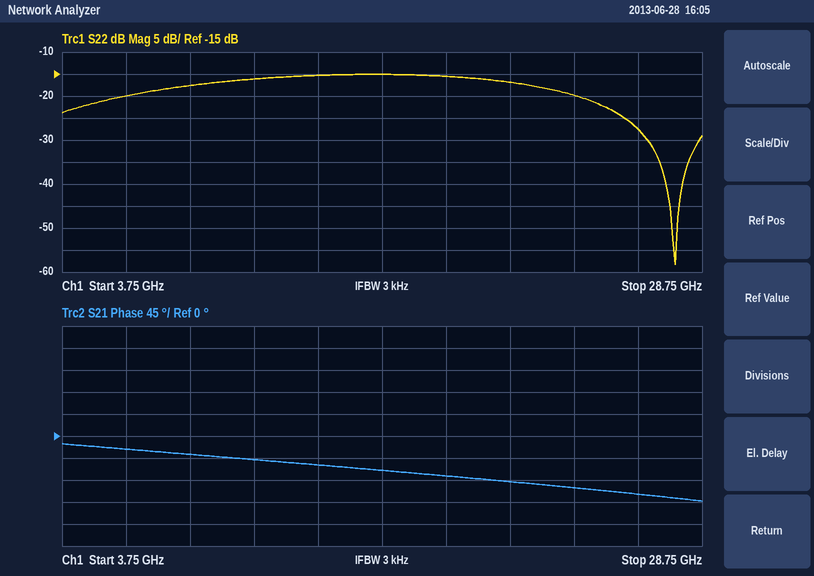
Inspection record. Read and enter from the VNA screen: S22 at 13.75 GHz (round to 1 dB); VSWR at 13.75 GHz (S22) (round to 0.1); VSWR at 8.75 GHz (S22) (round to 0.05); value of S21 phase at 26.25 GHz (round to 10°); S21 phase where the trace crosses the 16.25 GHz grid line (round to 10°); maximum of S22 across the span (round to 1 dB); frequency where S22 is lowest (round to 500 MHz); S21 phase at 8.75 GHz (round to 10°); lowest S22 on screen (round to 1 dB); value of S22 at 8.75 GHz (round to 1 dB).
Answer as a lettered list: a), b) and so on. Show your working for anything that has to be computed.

a) -15 dB
b) |Γ| = 10^(-15/20) = 0.1778; VSWR = (1 + 0.1778)/(1 − 0.1778) ≈ 1.4
c) |Γ| = 10^(-18/20) = 0.1259; VSWR = (1 + 0.1259)/(1 − 0.1259) ≈ 1.29, so 1.30 to the nearest 0.05
d) -120°
e) -70°
f) -15 dB
g) 27.5 GHz
h) -40°
i) -58 dB
j) -18 dB
